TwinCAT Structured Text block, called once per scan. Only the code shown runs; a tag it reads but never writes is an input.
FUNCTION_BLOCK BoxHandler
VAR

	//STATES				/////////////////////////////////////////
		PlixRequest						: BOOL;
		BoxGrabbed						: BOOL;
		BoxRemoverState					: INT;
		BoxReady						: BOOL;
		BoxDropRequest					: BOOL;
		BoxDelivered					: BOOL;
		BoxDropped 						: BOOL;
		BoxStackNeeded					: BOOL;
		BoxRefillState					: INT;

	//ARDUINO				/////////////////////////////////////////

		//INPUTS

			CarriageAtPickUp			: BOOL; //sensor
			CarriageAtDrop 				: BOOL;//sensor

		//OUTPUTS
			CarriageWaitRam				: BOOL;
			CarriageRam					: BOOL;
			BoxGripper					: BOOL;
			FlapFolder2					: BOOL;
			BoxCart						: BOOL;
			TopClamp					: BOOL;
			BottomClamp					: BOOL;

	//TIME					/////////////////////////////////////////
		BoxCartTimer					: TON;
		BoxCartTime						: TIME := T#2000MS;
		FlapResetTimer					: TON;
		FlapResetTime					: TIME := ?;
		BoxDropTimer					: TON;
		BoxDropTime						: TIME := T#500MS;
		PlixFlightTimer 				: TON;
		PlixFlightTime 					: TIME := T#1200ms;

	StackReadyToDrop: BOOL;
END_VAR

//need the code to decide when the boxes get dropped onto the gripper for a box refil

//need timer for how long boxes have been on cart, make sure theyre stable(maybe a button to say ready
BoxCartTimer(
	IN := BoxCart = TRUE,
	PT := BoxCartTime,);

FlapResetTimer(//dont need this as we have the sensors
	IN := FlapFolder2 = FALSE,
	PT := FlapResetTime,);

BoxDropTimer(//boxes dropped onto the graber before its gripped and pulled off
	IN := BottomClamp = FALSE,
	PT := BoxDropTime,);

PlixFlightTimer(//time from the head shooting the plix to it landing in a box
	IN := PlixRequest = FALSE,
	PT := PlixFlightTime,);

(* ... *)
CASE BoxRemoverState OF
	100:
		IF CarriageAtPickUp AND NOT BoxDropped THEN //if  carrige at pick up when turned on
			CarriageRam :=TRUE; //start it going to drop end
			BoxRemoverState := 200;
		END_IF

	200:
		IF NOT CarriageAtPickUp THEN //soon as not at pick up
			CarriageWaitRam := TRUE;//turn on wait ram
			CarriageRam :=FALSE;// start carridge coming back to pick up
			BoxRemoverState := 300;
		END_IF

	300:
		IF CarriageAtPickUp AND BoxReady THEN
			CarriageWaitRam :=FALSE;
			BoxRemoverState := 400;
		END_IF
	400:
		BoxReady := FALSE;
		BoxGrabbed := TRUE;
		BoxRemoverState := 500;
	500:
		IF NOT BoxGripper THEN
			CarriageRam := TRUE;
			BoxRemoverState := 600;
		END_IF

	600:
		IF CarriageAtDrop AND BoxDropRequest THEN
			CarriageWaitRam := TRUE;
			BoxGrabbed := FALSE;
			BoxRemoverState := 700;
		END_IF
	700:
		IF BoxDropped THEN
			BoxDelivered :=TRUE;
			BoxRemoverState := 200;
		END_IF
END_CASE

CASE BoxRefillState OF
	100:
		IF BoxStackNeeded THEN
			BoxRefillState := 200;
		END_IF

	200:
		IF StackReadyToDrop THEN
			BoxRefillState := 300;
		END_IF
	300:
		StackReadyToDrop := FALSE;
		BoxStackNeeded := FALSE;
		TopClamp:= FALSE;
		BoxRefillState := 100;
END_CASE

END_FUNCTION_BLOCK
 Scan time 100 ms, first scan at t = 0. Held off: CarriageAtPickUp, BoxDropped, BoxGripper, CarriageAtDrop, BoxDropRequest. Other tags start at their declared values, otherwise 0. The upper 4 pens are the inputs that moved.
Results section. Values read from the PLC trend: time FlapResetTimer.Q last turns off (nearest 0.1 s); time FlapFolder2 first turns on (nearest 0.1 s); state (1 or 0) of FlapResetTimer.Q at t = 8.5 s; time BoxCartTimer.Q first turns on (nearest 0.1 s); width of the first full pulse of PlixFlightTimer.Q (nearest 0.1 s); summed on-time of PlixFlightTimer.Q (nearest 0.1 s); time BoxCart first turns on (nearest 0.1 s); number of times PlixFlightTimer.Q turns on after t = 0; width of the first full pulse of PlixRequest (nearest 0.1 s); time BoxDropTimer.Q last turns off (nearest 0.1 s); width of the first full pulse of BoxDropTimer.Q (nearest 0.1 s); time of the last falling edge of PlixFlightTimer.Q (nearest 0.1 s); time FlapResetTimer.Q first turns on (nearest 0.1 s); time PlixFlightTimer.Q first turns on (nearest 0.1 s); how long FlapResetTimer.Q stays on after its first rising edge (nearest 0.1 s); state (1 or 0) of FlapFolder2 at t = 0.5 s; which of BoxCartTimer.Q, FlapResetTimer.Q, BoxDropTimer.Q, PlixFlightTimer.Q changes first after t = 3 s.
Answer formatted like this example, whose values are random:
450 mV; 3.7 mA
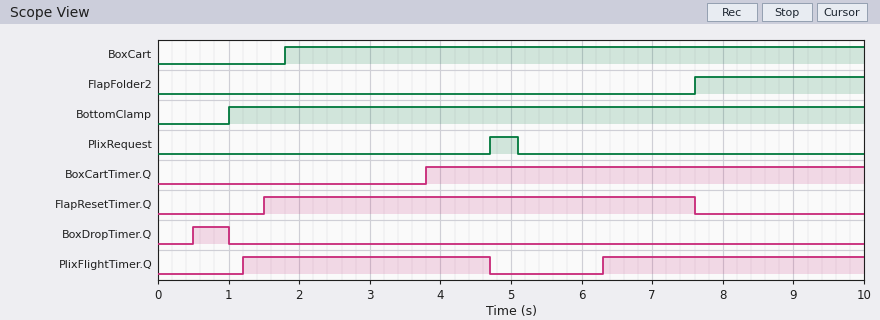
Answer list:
7.6 s; 7.6 s; 0; 3.8 s; 3.5 s; 7.2 s; 1.8 s; 2; 0.4 s; 1.0 s; 0.5 s; 4.7 s; 1.5 s; 1.2 s; 6.1 s; 0; BoxCartTimer.Q
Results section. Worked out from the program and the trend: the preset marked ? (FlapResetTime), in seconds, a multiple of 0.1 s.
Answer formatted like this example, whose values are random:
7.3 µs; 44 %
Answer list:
1.5 s
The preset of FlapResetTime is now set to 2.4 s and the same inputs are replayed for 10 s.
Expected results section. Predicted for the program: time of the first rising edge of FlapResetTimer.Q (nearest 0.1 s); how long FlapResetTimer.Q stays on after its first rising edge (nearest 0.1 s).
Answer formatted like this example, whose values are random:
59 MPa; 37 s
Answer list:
2.4 s; 5.2 s
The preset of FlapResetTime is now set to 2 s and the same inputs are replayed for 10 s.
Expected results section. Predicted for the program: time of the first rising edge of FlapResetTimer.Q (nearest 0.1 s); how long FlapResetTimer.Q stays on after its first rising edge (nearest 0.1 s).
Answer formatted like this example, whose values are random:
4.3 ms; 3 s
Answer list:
2.0 s; 5.6 s
